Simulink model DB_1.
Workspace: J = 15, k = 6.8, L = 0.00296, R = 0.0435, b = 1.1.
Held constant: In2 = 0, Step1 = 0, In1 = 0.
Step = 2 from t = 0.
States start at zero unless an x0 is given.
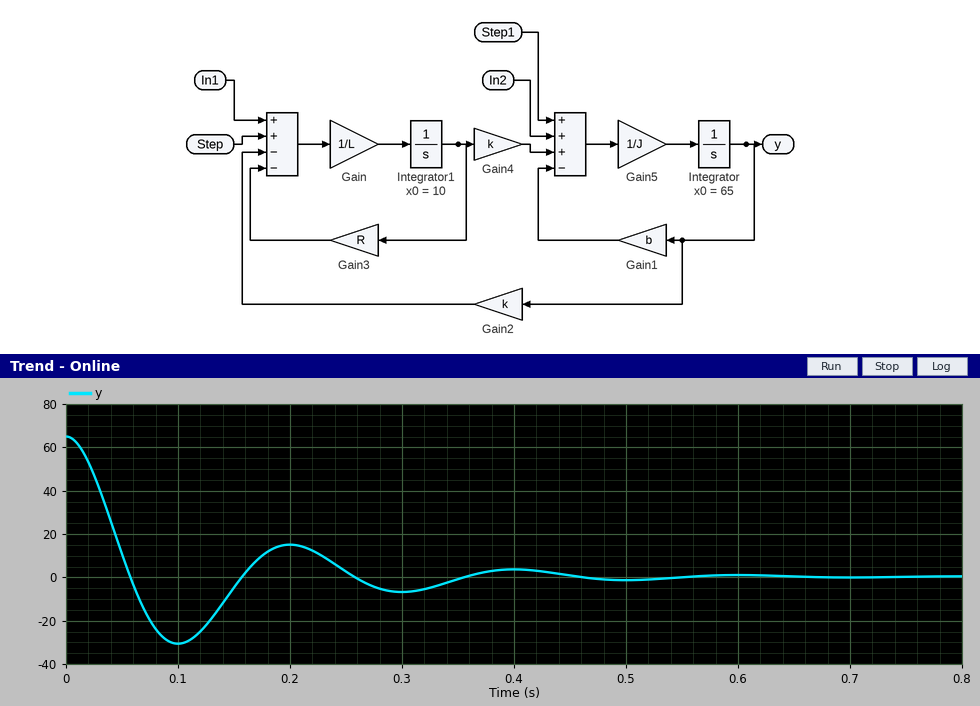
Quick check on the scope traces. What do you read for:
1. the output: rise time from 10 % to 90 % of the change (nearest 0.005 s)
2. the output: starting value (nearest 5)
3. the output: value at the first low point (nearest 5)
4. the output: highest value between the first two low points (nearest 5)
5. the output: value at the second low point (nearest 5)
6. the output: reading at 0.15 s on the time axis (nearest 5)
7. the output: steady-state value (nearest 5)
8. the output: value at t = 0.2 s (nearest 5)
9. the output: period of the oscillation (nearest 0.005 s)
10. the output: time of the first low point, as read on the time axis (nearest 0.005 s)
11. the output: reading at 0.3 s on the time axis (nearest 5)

0.040 s
65
-30
15
-5
-5
0
15
0.200 s
0.100 s
-5
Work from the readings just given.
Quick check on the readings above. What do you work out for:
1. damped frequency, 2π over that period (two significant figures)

31 rad/s
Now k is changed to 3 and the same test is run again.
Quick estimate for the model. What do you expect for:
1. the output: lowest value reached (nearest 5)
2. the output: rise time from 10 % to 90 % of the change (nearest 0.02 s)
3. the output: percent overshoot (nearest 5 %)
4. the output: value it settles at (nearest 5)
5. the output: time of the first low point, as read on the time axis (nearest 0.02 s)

-10
0.12 s
15 %
0
0.26 s
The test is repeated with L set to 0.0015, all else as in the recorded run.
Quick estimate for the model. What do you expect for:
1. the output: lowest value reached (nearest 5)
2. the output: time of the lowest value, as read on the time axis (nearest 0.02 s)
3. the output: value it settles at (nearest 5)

-20
0.08 s
0
